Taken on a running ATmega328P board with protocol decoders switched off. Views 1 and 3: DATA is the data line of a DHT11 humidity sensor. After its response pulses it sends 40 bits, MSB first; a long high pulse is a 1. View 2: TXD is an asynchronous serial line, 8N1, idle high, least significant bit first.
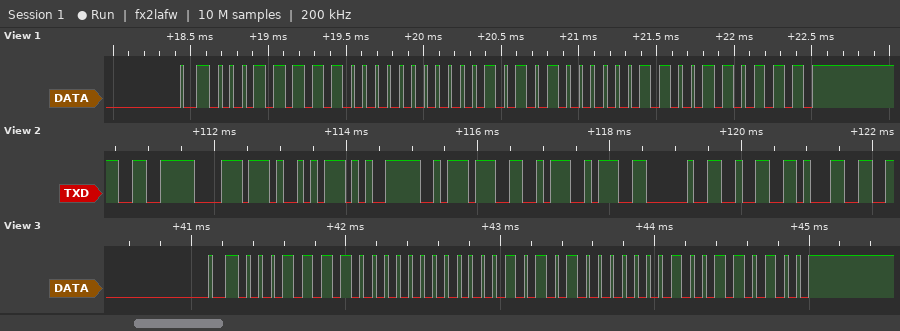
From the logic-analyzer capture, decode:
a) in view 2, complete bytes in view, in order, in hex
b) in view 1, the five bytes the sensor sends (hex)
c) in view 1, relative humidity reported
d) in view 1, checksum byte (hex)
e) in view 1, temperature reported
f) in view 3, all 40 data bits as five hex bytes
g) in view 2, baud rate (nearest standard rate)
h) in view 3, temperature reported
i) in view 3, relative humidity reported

E6 B8 A9 E5 BA A6 3A 20 32 31
1F 00 15 03 37
31 %
0x37
21.3 °C
1E 00 15 01 34
9600 baud
21.1 °C
30 %
